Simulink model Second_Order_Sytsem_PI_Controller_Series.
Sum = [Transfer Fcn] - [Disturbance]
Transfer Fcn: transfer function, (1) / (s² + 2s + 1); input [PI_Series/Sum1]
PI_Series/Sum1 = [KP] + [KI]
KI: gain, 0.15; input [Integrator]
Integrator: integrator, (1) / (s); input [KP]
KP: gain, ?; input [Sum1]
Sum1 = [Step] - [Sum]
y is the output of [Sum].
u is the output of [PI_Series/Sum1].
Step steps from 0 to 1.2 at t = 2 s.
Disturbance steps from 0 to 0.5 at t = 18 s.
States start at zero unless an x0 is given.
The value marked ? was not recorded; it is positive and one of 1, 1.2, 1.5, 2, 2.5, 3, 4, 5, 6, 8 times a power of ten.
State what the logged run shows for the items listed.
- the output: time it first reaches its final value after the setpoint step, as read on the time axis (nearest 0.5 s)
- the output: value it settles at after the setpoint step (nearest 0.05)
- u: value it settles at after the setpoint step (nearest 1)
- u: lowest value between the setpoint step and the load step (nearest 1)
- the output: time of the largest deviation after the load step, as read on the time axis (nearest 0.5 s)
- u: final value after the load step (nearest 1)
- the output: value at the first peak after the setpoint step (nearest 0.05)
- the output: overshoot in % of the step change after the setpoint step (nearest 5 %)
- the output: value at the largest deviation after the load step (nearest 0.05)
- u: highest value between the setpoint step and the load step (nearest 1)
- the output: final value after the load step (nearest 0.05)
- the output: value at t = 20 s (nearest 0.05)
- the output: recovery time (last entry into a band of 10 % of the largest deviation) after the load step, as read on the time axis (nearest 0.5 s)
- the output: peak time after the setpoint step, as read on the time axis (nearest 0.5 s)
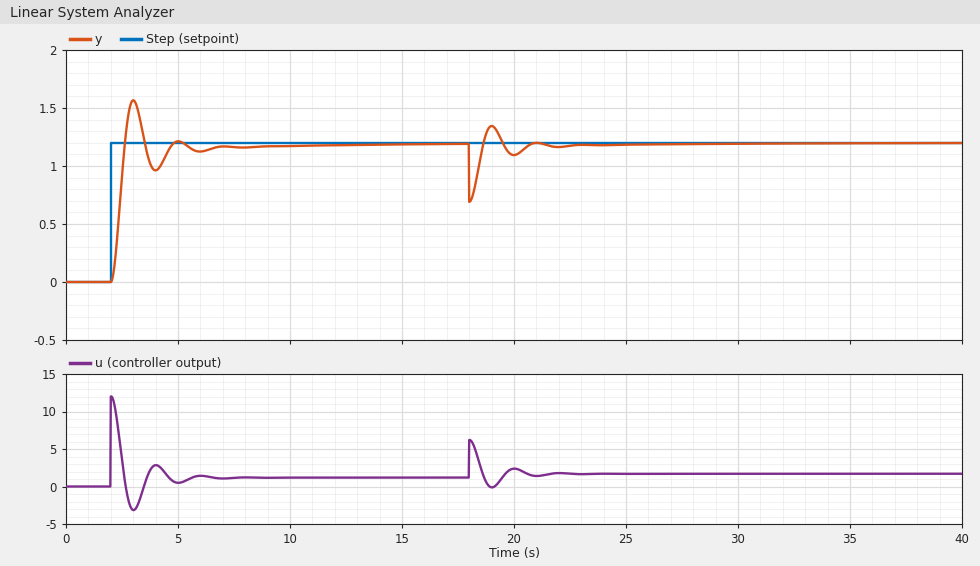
2.5 s
1.20
1
-3
18.0 s
2
1.55
30 %
0.70
12
1.20
1.10
20.5 s
3.0 s
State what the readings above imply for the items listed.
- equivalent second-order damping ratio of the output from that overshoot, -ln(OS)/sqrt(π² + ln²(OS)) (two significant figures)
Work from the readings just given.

0.36
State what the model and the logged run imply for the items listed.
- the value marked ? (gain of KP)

10
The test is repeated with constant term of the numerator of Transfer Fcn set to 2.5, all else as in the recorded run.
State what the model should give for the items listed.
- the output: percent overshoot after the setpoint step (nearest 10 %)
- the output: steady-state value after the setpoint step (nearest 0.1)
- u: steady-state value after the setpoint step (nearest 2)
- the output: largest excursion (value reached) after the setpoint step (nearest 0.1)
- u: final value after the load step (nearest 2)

50 %
1.2
0
1.8
0
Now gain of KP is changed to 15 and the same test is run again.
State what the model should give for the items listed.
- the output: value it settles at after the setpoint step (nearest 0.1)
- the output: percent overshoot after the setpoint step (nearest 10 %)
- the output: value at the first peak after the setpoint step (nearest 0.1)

1.2
40 %
1.7
